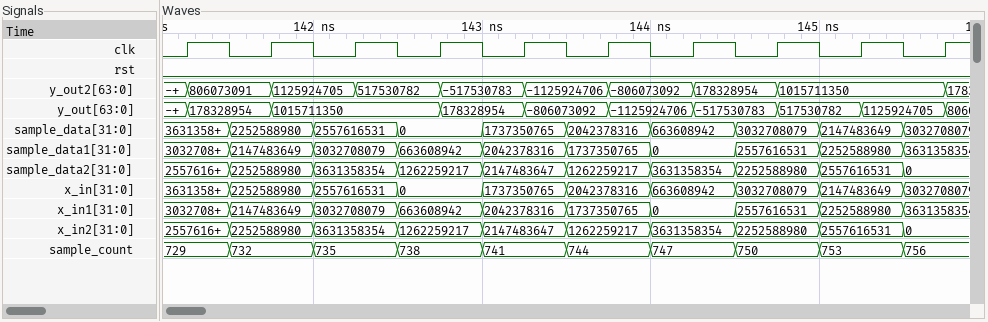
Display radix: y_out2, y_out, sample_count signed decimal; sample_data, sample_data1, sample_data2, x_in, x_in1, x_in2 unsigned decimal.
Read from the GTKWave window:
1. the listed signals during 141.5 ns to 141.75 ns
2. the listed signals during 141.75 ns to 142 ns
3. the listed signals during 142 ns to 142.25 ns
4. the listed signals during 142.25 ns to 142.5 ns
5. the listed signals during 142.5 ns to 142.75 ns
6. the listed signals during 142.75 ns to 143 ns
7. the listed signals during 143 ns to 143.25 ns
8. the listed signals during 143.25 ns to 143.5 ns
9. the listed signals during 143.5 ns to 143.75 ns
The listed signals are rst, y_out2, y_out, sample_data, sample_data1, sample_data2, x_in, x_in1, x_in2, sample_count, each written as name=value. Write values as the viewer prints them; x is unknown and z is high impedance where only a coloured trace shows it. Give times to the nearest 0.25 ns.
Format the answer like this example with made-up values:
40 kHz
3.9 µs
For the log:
rst=0, y_out2=806073091, y_out=178328954, sample_data=2252588980, sample_data1=2147483649, sample_data2=2252588980, x_in=2252588980, x_in1=2147483649, x_in2=2252588980, sample_count=732
rst=0, y_out2=1125924705, y_out=1015711350, sample_data=2252588980, sample_data1=2147483649, sample_data2=2252588980, x_in=2252588980, x_in1=2147483649, x_in2=2252588980, sample_count=732
rst=0, y_out2=1125924705, y_out=1015711350, sample_data=2557616531, sample_data1=3032708079, sample_data2=3631358354, x_in=2557616531, x_in1=3032708079, x_in2=3631358354, sample_count=735
rst=0, y_out2=517530782, y_out=1015711350, sample_data=2557616531, sample_data1=3032708079, sample_data2=3631358354, x_in=2557616531, x_in1=3032708079, x_in2=3631358354, sample_count=735
rst=0, y_out2=517530782, y_out=1015711350, sample_data=0, sample_data1=663608942, sample_data2=1262259217, x_in=0, x_in1=663608942, x_in2=1262259217, sample_count=738
rst=0, y_out2=-517530783, y_out=178328954, sample_data=0, sample_data1=663608942, sample_data2=1262259217, x_in=0, x_in1=663608942, x_in2=1262259217, sample_count=738
rst=0, y_out2=-517530783, y_out=178328954, sample_data=1737350765, sample_data1=2042378316, sample_data2=2147483647, x_in=1737350765, x_in1=2042378316, x_in2=2147483647, sample_count=741
rst=0, y_out2=-1125924706, y_out=-806073092, sample_data=1737350765, sample_data1=2042378316, sample_data2=2147483647, x_in=1737350765, x_in1=2042378316, x_in2=2147483647, sample_count=741
rst=0, y_out2=-1125924706, y_out=-806073092, sample_data=2042378316, sample_data1=1737350765, sample_data2=1262259217, x_in=2042378316, x_in1=1737350765, x_in2=1262259217, sample_count=744
